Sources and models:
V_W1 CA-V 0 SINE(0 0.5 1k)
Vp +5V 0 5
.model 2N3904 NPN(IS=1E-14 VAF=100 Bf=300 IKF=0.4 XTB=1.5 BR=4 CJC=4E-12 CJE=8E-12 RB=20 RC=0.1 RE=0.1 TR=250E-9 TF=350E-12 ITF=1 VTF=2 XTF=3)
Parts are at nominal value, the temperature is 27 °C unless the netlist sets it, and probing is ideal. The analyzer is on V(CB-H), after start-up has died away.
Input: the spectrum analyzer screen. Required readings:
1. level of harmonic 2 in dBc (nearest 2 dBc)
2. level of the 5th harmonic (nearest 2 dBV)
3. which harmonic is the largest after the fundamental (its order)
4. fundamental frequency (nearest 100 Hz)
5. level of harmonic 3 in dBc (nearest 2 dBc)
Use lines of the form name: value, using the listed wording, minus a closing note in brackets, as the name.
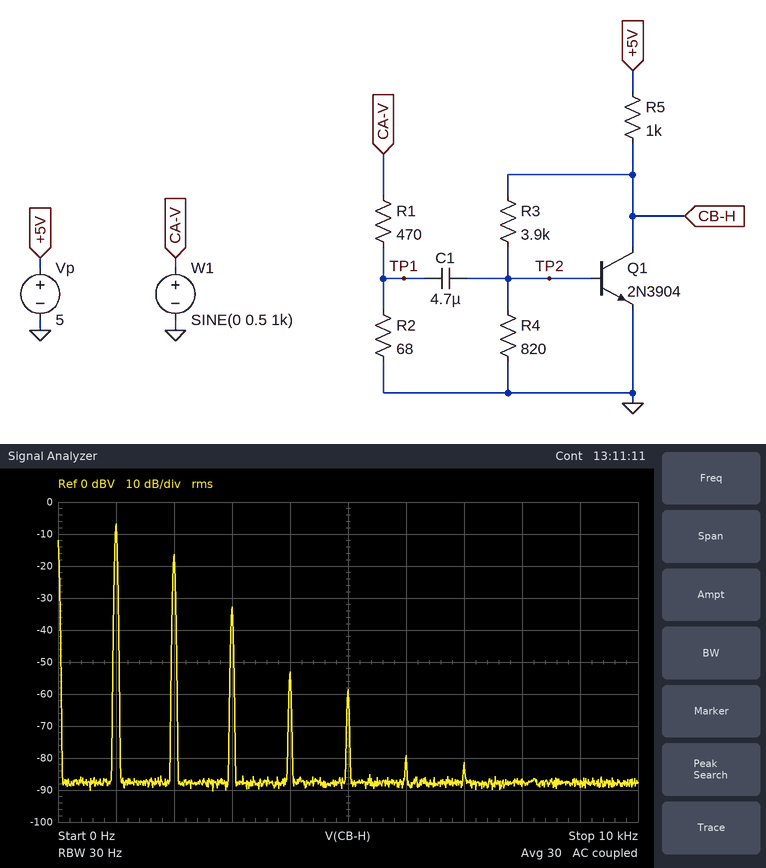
level of harmonic 2 in dBc: -10 dBc
level of the 5th harmonic: -58 dBV
which harmonic is the largest after the fundamental: 2
fundamental frequency: 1.0 kHz
level of harmonic 3 in dBc: -26 dBc
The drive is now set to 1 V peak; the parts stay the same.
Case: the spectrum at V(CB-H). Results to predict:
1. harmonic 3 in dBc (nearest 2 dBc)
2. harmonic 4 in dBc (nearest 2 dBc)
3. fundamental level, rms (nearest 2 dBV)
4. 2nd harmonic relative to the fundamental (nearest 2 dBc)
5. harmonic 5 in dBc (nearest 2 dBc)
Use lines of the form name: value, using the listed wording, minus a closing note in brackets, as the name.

harmonic 3 in dBc: -16 dBc
harmonic 4 in dBc: -38 dBc
fundamental level, rms: -2 dBV
2nd harmonic relative to the fundamental: -6 dBc
harmonic 5 in dBc: -36 dBc
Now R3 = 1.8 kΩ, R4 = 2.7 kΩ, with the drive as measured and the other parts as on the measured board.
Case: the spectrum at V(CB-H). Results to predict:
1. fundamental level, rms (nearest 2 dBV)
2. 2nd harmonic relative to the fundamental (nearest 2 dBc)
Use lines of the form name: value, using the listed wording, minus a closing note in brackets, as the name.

fundamental level, rms: -2 dBV
2nd harmonic relative to the fundamental: -46 dBc
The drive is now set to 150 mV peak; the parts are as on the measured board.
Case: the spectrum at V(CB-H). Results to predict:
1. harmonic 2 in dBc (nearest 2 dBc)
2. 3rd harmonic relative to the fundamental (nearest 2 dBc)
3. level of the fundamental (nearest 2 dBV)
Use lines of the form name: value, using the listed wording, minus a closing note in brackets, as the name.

harmonic 2 in dBc: -20 dBc
3rd harmonic relative to the fundamental: -48 dBc
level of the fundamental: -16 dBV
